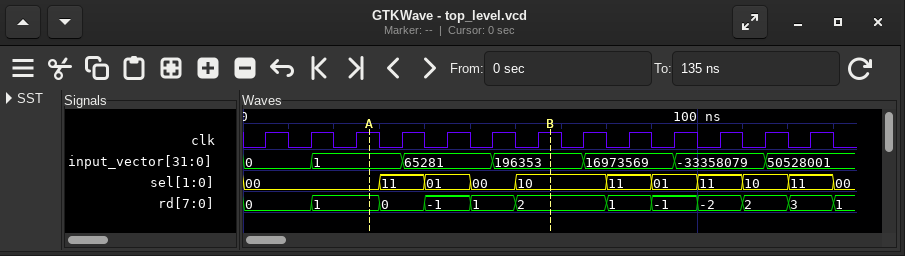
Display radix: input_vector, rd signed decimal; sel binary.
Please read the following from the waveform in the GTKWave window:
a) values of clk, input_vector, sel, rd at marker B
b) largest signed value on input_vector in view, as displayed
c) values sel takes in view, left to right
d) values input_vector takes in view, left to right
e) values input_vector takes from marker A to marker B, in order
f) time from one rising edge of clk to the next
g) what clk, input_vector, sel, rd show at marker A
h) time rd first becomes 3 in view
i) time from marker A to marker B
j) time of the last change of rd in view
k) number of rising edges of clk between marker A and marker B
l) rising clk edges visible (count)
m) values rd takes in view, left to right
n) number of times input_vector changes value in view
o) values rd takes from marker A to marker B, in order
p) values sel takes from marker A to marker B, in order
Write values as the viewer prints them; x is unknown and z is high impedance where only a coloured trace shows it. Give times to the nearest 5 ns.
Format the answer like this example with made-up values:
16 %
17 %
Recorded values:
clk=1, input_vector=196353, sel=10, rd=2
50528001
00, 11, 01, 00, 10, 11, 01, 11, 10, 11, 00
0, 1, 65281, 196353, 16973569, -33358079, 50528001
1, 65281, 196353
10 ns
clk=1, input_vector=1, sel=00, rd=1
120 ns
40 ns
130 ns
4
13
0, 1, 0, -1, 1, 2, 1, -1, -2, 2, 3, 1
6
1, 0, -1, 1, 2
00, 11, 01, 00, 10
